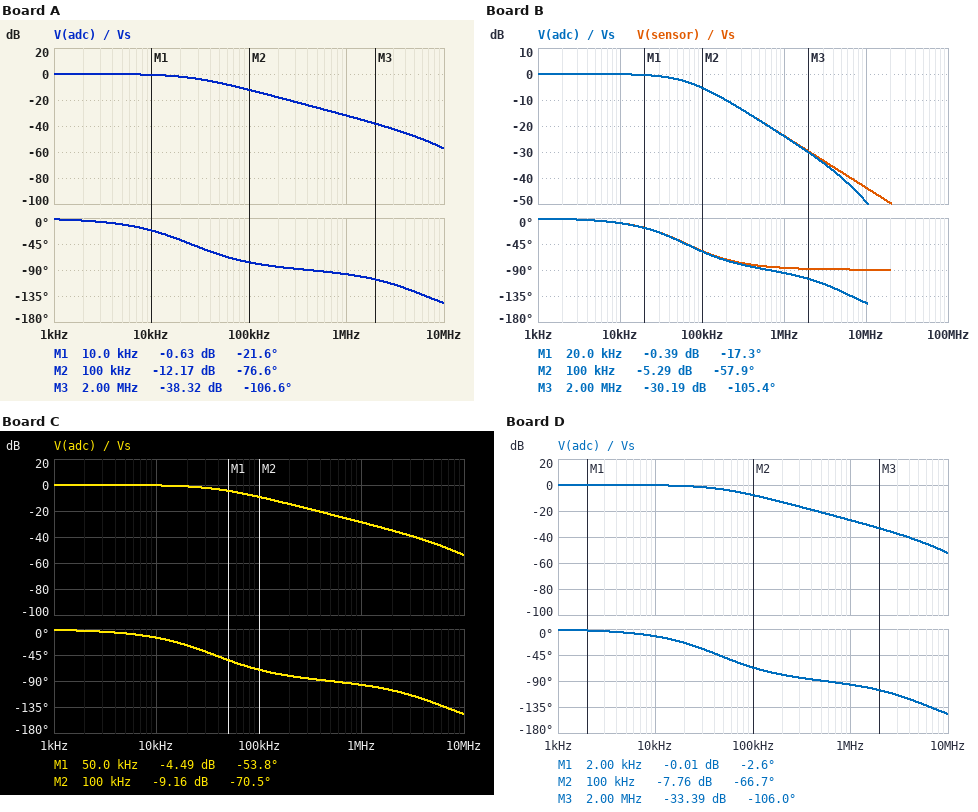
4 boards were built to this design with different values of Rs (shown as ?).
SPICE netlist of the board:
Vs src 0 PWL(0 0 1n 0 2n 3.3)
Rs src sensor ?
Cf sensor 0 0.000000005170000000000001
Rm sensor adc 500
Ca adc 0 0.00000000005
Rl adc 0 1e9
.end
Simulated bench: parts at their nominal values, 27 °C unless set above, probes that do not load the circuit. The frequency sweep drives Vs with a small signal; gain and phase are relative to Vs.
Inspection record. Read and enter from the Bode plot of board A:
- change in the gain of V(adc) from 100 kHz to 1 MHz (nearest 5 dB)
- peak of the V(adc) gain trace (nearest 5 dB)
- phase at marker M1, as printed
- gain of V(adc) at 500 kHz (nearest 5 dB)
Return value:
-20 dB
0 dB
-21.6 deg
-25 dB
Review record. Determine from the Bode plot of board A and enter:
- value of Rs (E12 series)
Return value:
1.2 kΩ
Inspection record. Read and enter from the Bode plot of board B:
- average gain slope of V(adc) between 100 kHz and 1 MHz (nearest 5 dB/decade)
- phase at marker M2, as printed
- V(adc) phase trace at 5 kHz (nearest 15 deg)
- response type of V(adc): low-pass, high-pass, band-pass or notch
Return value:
-20 dB/decade
-57.9 deg
0 deg
low-pass
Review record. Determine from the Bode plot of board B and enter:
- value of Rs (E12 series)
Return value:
470 Ω
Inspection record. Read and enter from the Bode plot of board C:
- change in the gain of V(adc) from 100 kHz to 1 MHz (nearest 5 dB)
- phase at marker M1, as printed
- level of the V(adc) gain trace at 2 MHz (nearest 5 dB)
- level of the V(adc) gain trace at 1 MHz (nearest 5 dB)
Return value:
-20 dB
-53.8 deg
-35 dB
-30 dB
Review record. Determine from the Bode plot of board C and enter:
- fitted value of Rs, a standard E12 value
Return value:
820 Ω
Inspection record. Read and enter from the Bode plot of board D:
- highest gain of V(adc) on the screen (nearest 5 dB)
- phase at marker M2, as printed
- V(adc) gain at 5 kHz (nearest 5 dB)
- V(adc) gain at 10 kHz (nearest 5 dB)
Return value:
0 dB
-66.7 deg
0 dB
0 dB
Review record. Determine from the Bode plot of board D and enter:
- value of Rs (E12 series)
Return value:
680 Ω
